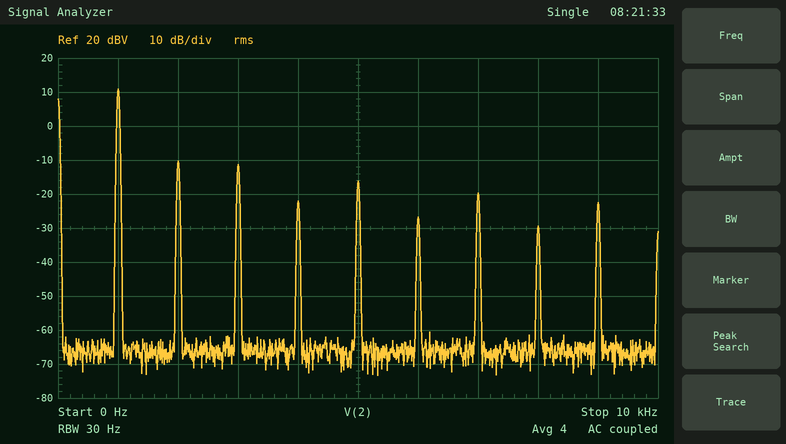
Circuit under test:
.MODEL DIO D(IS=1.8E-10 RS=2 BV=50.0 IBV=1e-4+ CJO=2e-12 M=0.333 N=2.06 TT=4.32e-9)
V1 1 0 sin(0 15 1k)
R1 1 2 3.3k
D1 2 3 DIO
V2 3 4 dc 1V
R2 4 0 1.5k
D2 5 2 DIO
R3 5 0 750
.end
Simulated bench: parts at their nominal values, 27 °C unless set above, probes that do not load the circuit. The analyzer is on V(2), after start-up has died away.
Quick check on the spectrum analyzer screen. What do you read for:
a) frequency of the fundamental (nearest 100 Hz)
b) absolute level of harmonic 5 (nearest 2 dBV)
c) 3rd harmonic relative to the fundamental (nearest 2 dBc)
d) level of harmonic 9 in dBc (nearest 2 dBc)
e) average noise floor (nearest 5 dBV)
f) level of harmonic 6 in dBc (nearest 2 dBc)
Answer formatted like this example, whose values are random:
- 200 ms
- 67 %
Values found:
- 1.0 kHz
- -16 dBV
- -22 dBc
- -34 dBc
- -65 dBV
- -38 dBc
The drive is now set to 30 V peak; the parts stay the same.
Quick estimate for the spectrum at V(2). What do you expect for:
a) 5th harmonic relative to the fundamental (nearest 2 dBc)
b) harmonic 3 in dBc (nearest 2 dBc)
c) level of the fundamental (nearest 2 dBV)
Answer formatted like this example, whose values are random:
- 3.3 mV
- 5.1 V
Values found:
- -32 dBc
- -26 dBc
- 16 dBV
